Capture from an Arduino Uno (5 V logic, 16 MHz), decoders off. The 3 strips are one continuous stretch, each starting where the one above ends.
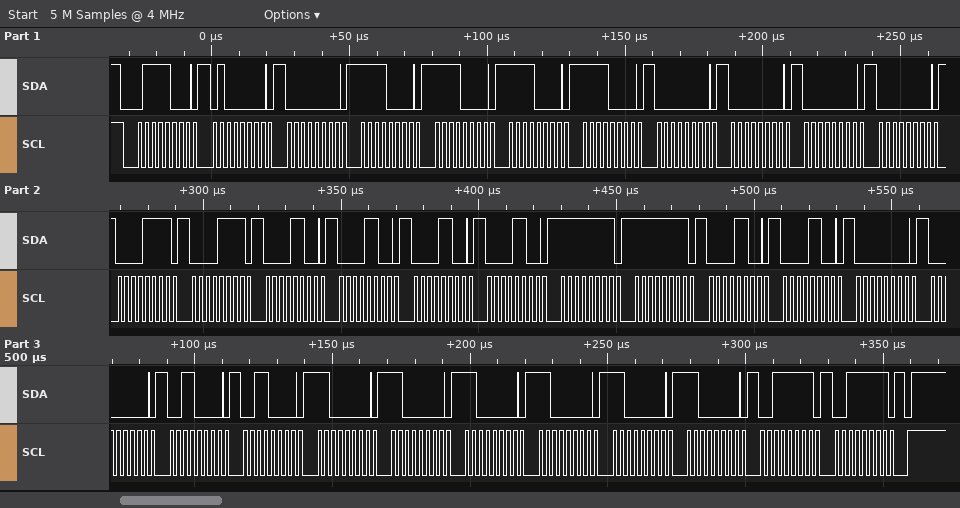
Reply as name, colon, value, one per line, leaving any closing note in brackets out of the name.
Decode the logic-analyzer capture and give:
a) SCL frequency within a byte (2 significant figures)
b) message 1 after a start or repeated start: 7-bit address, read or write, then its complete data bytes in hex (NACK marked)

SCL frequency within a byte: 400 kHz
message 1 after a start or repeated start: 7-bit address, read or write, then its complete data bytes in hex: 0x3C write: 40 00 F0 F0 F0 F0 00 00 00 00 0F 0F 0C 0C 0C 0C FF FF 0C 0C 00 00 30 30 C0 C0 C0 C0 C0 C0 3F 3F
